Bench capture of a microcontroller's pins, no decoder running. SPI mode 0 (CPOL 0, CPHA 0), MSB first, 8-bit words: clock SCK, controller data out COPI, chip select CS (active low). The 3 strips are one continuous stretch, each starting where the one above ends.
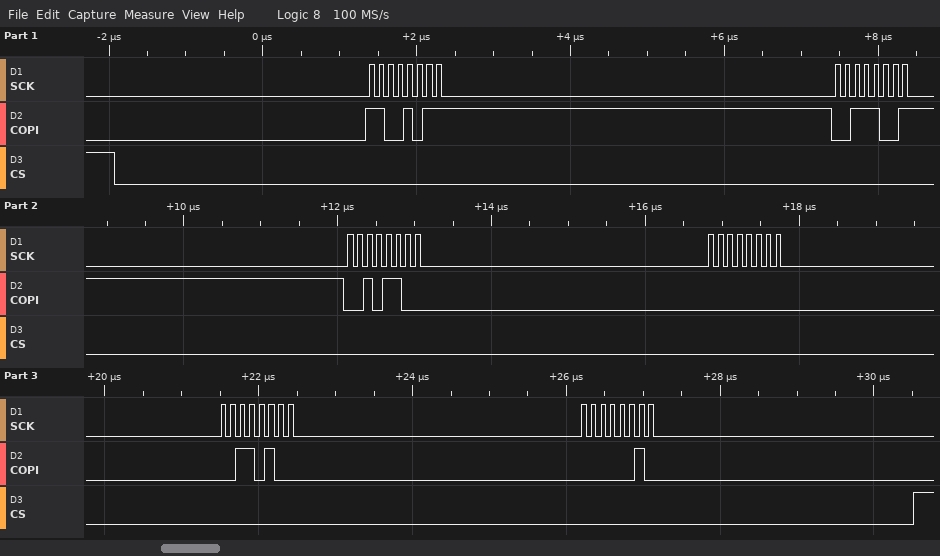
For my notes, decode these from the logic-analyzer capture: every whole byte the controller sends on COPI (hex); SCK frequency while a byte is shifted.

CB 39 2C 00 34 02
8 MHz
